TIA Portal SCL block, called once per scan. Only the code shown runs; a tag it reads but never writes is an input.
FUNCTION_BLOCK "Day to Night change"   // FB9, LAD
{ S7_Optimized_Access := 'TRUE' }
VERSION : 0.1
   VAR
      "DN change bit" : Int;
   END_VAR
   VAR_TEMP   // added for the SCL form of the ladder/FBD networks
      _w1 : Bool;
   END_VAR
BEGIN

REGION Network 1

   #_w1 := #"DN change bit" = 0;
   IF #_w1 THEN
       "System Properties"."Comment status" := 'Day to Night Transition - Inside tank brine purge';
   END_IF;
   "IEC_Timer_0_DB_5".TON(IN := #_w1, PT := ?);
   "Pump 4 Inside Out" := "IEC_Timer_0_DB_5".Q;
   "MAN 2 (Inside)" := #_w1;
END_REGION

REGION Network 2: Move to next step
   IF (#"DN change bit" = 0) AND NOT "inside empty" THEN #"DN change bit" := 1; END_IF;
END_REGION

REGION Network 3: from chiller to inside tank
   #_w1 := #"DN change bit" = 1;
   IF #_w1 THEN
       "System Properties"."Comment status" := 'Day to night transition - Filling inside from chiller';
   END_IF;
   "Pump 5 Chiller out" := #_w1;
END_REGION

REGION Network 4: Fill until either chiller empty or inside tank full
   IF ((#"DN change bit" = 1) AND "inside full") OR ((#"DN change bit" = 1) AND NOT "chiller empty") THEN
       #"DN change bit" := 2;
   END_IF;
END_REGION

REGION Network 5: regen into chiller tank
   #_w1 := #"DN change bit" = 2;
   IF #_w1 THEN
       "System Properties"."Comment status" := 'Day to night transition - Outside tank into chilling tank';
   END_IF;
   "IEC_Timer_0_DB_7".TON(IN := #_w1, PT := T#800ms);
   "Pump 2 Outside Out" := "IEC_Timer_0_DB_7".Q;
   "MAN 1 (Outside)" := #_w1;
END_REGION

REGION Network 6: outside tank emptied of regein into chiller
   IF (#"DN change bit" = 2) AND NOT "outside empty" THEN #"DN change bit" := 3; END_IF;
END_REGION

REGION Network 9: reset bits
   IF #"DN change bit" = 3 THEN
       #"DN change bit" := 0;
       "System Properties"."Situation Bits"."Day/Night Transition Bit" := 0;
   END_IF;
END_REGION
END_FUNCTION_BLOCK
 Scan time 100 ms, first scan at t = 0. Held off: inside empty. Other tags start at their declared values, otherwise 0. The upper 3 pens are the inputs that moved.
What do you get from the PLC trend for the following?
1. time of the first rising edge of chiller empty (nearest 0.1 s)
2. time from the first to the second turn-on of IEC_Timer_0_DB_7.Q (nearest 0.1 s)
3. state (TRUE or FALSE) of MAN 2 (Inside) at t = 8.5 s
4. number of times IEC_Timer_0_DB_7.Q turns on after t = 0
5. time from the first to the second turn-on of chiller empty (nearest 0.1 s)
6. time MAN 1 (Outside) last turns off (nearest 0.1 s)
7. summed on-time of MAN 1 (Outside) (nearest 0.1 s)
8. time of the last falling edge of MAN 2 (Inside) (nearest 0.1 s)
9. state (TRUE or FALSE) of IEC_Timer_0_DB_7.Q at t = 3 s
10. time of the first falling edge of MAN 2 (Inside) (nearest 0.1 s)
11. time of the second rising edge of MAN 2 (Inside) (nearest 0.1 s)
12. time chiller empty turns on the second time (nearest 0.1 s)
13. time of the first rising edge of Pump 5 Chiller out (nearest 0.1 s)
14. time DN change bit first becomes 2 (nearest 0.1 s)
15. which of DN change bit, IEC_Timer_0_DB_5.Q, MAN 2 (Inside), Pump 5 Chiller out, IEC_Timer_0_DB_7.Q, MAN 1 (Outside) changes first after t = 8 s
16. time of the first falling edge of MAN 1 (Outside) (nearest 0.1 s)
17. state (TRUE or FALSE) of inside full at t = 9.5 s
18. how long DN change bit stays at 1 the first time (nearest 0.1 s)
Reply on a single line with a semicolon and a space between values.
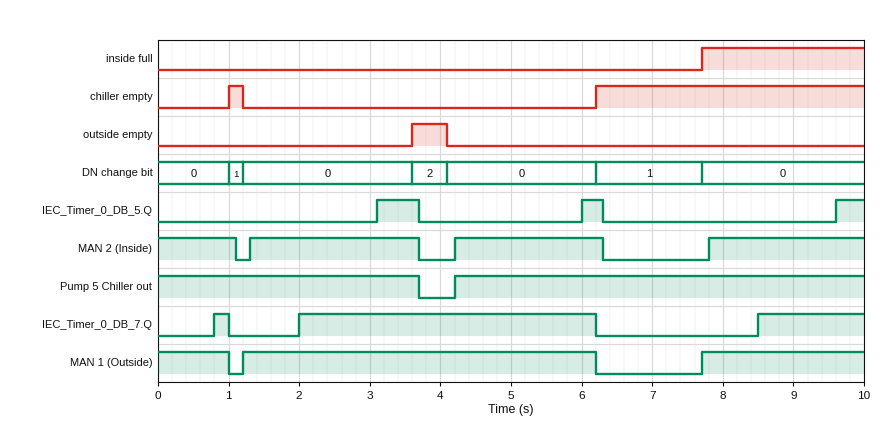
1.0 s; 1.2 s; TRUE; 3; 5.2 s; 6.2 s; 8.3 s; 6.3 s; TRUE; 1.1 s; 4.2 s; 6.2 s; 4.2 s; 3.6 s; IEC_Timer_0_DB_7.Q; 1.0 s; TRUE; 0.2 s
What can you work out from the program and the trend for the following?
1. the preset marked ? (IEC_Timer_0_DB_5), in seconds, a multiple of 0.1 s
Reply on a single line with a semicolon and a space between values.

1.8 s
